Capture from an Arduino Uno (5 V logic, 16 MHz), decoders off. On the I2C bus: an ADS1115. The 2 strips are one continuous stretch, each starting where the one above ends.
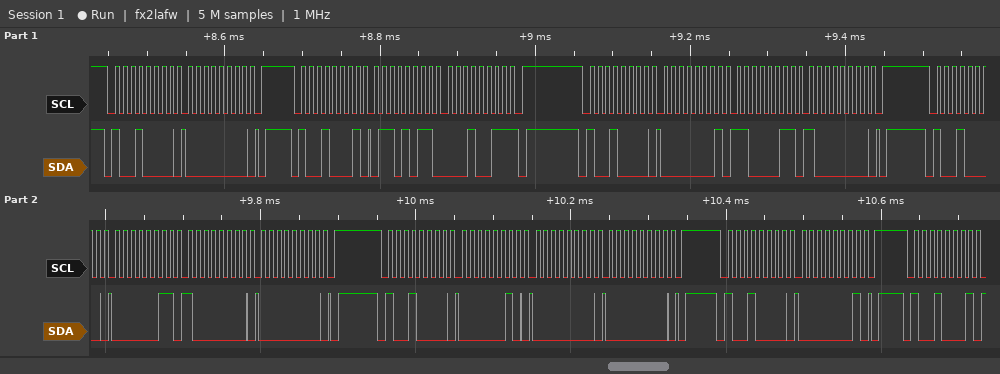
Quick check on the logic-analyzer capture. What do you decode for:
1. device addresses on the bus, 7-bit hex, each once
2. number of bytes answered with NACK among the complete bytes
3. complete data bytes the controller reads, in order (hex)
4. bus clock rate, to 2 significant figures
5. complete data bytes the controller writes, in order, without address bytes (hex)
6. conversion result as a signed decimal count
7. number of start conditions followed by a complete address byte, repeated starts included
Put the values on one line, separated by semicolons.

0x48; 1; 6B 13; 100 kHz; 00 01 C3 80 03 80 00 02 00 00 01; 27411; 7
